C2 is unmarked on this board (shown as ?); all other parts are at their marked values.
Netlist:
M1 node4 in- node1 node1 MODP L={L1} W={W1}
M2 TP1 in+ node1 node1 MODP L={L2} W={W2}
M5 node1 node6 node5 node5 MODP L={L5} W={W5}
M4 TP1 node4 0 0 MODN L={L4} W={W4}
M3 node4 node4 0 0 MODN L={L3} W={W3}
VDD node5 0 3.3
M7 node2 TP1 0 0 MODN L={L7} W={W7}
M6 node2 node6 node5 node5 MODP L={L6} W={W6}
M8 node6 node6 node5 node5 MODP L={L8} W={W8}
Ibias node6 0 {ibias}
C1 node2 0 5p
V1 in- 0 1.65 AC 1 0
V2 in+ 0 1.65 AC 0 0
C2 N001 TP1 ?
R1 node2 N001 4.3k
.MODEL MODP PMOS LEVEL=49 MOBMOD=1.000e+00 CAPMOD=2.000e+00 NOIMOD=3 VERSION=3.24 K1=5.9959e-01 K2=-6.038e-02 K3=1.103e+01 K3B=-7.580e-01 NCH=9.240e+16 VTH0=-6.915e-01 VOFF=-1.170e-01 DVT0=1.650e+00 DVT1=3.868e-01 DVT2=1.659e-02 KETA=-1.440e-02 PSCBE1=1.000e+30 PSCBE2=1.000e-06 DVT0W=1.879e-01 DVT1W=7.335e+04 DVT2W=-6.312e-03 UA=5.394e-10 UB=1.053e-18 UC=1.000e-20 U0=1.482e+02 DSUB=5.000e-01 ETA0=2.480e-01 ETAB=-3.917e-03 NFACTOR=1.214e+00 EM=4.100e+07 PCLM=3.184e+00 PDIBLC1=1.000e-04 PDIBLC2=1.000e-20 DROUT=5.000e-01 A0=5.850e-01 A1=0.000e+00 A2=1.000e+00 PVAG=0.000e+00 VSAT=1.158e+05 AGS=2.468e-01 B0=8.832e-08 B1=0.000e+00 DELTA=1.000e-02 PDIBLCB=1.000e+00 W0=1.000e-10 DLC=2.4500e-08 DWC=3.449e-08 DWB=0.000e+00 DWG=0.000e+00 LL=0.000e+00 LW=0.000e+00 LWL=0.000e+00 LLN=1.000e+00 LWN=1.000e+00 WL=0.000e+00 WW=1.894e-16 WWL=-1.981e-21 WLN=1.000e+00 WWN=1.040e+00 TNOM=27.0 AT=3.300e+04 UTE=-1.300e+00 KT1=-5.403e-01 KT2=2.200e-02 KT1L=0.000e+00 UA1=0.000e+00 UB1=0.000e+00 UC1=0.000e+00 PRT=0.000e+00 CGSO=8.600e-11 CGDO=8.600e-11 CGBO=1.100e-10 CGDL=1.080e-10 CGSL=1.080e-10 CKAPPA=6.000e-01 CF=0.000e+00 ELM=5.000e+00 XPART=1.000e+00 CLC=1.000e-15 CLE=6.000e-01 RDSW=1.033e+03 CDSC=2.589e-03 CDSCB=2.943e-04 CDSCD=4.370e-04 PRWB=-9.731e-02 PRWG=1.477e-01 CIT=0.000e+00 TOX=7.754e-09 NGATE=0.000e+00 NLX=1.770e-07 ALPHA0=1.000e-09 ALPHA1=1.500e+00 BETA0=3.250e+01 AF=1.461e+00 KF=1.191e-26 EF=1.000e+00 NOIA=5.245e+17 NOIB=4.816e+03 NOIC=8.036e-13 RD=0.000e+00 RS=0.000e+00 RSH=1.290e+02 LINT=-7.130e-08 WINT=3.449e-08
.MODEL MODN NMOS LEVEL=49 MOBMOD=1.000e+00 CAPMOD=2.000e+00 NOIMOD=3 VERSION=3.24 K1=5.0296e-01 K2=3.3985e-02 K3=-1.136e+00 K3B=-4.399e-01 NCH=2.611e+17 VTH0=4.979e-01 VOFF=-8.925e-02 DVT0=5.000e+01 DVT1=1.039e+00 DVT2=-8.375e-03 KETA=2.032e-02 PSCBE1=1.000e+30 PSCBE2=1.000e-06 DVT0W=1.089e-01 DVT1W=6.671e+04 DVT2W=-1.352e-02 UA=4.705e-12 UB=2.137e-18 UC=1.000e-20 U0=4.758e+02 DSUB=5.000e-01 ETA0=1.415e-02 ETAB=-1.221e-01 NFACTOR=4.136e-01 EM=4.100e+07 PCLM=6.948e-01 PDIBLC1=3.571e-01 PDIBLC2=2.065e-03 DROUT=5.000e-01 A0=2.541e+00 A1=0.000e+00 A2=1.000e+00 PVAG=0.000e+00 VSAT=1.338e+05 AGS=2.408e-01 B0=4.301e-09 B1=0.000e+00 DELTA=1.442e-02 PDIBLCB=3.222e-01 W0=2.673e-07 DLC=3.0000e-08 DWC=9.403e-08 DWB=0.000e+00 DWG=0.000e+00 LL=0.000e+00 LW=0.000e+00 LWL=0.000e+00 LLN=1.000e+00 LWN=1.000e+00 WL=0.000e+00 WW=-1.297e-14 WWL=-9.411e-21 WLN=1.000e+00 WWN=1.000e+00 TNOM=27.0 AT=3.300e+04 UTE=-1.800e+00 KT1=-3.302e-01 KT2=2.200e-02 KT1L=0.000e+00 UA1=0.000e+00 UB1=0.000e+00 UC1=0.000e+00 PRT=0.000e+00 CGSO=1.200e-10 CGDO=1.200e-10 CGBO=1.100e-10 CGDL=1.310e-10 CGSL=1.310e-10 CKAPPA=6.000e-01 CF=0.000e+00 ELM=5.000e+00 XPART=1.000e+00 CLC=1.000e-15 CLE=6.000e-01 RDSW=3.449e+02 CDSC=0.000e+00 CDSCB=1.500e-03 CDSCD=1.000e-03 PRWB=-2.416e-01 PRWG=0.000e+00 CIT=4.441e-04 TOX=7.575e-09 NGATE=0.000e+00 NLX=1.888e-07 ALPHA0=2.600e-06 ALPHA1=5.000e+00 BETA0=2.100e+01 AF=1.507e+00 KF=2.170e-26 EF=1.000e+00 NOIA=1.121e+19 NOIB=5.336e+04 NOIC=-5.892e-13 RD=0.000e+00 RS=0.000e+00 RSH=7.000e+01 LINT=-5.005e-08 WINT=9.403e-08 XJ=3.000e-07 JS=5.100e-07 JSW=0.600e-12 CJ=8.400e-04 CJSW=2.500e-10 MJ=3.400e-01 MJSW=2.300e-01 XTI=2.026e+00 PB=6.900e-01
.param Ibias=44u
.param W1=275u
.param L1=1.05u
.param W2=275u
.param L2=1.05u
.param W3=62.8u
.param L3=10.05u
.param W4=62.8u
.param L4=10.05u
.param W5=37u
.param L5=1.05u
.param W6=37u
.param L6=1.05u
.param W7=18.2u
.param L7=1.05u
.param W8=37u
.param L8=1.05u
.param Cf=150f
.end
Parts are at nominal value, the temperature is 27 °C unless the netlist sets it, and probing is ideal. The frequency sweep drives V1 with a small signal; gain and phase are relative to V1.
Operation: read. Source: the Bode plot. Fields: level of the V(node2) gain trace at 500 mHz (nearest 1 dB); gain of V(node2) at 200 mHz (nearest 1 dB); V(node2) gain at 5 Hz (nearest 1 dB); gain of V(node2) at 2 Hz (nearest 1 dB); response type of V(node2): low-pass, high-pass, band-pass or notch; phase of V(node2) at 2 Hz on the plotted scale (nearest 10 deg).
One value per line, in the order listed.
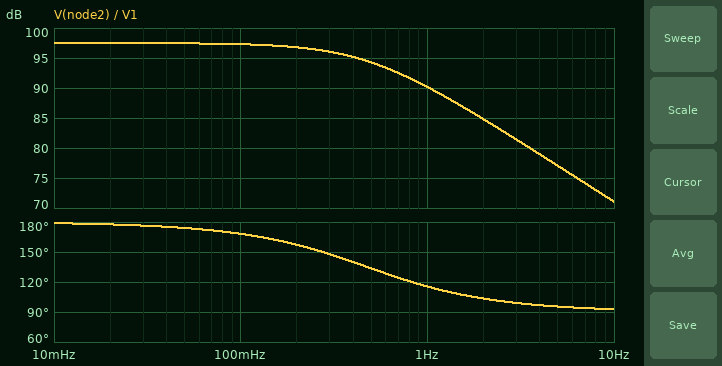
94 dB
97 dB
77 dB
85 dB
low-pass
100 deg
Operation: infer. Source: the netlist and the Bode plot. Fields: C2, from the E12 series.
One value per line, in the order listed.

1.8 nF
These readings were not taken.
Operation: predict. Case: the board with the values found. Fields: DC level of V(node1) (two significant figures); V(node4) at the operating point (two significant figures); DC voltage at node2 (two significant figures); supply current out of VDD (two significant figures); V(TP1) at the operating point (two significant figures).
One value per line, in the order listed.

2.4 V
720 mV
1.9 V
130 µA
720 mV
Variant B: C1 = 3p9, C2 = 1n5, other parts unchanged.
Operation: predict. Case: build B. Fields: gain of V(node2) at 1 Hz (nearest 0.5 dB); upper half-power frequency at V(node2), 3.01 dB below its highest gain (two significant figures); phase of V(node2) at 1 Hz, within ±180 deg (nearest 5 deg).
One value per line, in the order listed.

91.5 dB
570 mHz
120 deg
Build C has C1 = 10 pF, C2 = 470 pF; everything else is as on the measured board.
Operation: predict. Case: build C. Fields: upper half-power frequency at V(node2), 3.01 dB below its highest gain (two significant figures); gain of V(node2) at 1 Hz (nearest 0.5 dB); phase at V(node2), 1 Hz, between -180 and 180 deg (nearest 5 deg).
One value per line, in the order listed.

1.8 Hz
96.5 dB
150 deg
